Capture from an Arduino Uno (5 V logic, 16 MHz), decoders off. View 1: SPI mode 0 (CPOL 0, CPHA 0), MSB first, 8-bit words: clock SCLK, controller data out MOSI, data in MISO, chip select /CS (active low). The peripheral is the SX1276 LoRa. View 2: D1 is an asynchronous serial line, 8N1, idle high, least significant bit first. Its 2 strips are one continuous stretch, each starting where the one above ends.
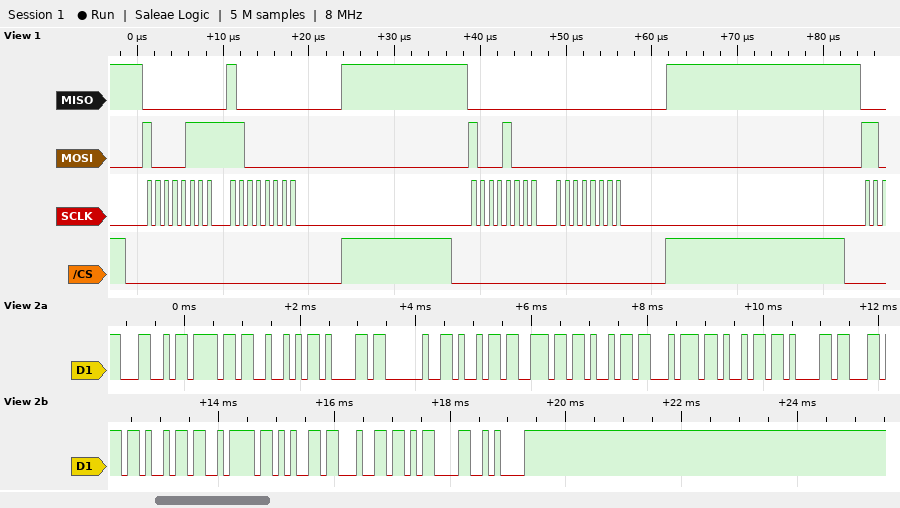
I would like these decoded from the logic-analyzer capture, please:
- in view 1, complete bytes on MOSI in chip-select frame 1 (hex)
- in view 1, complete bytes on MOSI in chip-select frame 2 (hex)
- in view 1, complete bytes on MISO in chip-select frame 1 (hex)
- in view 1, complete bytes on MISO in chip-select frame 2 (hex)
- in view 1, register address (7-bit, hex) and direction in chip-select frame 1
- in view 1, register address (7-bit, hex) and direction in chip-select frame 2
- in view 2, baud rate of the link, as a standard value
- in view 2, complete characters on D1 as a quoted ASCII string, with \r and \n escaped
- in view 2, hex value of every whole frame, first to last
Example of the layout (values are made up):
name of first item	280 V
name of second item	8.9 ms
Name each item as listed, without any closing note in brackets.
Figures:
in view 1, complete bytes on MOSI in chip-select frame 1	0x87 0xC0
in view 1, complete bytes on MOSI in chip-select frame 2	0x88 0x00
in view 1, complete bytes on MISO in chip-select frame 1	0x00 0x80
in view 1, complete bytes on MISO in chip-select frame 2	0x00 0x00
in view 1, register address (7-bit, hex) and direction in chip-select frame 1	0x07 write
in view 1, register address (7-bit, hex) and direction in chip-select frame 2	0x08 write
in view 2, baud rate of the link, as a standard value	9600 baud
in view 2, complete characters on D1 as a quoted ASCII string, with \r and \n escaped	"LoRa initialized\r\n"
in view 2, hex value of every whole frame, first to last	0x4C 0x6F 0x52 0x61 0x20 0x69 0x6E 0x69 0x74 0x69 0x61 0x6C 0x69 0x7A 0x65 0x64 0x0D 0x0A
